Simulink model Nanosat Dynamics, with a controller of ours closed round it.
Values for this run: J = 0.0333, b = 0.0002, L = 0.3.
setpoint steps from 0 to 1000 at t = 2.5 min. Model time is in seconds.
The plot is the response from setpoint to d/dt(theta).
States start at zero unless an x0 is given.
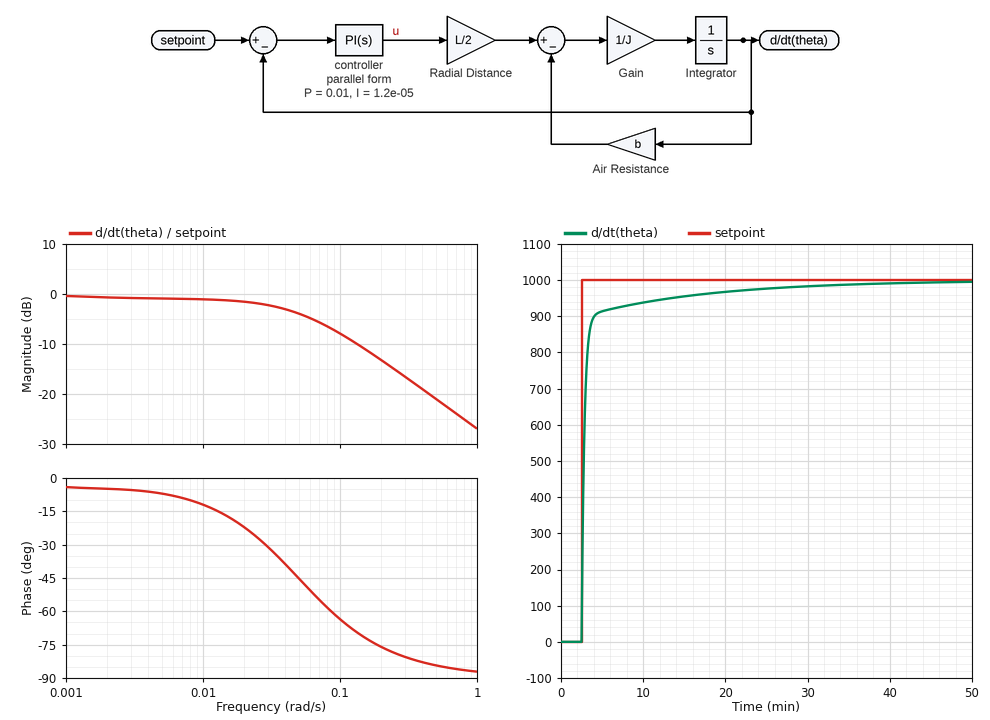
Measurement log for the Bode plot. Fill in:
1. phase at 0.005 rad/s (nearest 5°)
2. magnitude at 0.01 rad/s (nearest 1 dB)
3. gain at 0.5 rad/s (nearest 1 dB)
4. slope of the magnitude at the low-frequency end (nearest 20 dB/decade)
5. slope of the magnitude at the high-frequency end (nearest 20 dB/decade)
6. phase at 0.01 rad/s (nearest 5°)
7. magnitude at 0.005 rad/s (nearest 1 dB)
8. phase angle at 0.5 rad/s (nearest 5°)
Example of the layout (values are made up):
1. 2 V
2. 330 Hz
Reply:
1. -5°
2. -1 dB
3. -21 dB
4. 0 dB/decade
5. -20 dB/decade
6. -10°
7. -1 dB
8. -85°
